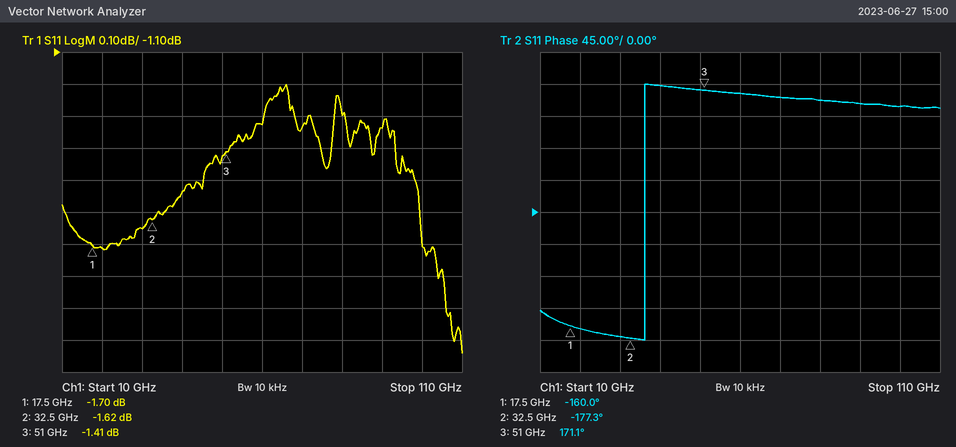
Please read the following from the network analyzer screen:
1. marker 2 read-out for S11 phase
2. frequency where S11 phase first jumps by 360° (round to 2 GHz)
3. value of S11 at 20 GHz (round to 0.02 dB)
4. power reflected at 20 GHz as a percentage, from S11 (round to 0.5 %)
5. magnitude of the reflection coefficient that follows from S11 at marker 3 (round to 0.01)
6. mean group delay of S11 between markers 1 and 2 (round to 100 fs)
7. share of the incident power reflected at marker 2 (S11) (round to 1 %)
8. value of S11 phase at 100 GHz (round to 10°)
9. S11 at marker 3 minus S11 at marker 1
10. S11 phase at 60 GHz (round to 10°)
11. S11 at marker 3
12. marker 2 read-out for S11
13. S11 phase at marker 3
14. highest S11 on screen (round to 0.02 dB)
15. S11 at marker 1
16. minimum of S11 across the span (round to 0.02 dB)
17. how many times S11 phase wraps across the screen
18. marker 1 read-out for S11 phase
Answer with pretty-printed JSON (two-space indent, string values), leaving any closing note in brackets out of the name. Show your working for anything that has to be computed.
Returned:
{
  "marker 2 read-out for S11 phase": "-177.3°",
  "frequency where S11 phase first jumps by 360°": "36 GHz",
  "value of S11 at 20 GHz": "-1.72 dB",
  "power reflected at 20 GHz as a percentage, from S11": "10^(-1.72/10) ≈ 67.3 %, so 67.5 % to the nearest 0.5 %",
  "magnitude of the reflection coefficient that follows from S11 at marker 3": "10^(-1.41/20) ≈ 0.85",
  "mean group delay of S11 between markers 1 and 2": "−(-177.3° − (-160°))/(360° × 15 GHz) ≈ 3.2 ps",
  "share of the incident power reflected at marker 2 (S11)": "10^(-1.62/10) ≈ 69 %",
  "value of S11 phase at 100 GHz": "150°",
  "S11 at marker 3 minus S11 at marker 1": "-1.41 − (-1.7) = 0.29 dB",
  "S11 phase at 60 GHz": "170°",
  "S11 at marker 3": "-1.41 dB",
  "marker 2 read-out for S11": "-1.62 dB",
  "S11 phase at marker 3": "171.1°",
  "highest S11 on screen": "-1.20 dB",
  "S11 at marker 1": "-1.70 dB",
  "minimum of S11 across the span": "-2.04 dB",
  "how many times S11 phase wraps across the screen": "1",
  "marker 1 read-out for S11 phase": "-160.0°"
}
